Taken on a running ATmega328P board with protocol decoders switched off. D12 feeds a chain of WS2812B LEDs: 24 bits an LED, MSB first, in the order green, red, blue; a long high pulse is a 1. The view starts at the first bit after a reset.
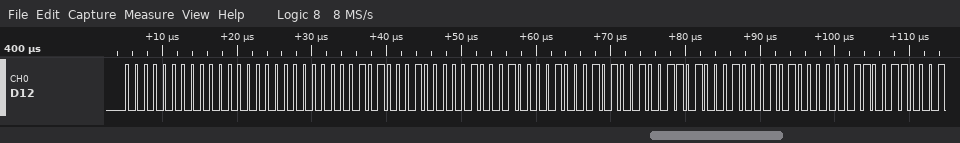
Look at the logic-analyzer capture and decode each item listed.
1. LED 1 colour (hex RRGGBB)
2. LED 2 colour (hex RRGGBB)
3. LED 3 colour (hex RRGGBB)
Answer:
#000000
#045142
#342945
